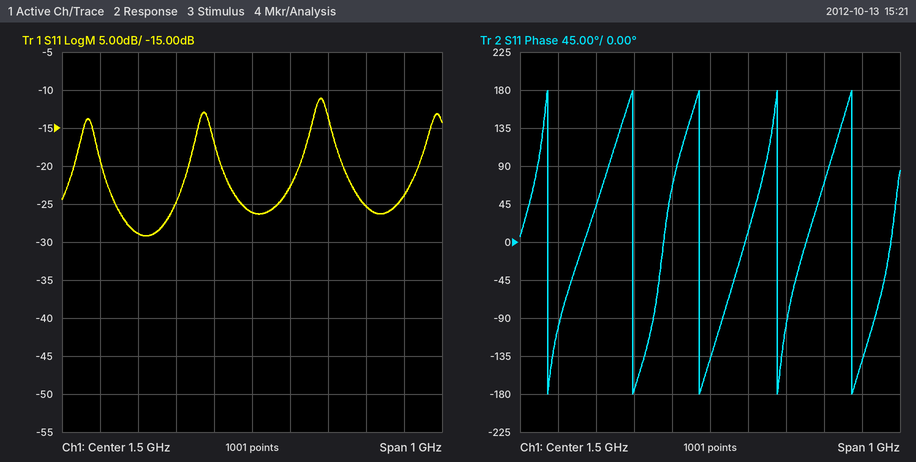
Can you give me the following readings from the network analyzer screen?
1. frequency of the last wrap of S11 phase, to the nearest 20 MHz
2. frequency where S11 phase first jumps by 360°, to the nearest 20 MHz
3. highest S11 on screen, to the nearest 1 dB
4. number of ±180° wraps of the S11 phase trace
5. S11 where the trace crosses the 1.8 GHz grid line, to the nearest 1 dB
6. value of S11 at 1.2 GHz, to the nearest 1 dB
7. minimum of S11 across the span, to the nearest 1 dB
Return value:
1.88 GHz
1.08 GHz
-11 dB
5
-25 dB
-29 dB
-29 dB
